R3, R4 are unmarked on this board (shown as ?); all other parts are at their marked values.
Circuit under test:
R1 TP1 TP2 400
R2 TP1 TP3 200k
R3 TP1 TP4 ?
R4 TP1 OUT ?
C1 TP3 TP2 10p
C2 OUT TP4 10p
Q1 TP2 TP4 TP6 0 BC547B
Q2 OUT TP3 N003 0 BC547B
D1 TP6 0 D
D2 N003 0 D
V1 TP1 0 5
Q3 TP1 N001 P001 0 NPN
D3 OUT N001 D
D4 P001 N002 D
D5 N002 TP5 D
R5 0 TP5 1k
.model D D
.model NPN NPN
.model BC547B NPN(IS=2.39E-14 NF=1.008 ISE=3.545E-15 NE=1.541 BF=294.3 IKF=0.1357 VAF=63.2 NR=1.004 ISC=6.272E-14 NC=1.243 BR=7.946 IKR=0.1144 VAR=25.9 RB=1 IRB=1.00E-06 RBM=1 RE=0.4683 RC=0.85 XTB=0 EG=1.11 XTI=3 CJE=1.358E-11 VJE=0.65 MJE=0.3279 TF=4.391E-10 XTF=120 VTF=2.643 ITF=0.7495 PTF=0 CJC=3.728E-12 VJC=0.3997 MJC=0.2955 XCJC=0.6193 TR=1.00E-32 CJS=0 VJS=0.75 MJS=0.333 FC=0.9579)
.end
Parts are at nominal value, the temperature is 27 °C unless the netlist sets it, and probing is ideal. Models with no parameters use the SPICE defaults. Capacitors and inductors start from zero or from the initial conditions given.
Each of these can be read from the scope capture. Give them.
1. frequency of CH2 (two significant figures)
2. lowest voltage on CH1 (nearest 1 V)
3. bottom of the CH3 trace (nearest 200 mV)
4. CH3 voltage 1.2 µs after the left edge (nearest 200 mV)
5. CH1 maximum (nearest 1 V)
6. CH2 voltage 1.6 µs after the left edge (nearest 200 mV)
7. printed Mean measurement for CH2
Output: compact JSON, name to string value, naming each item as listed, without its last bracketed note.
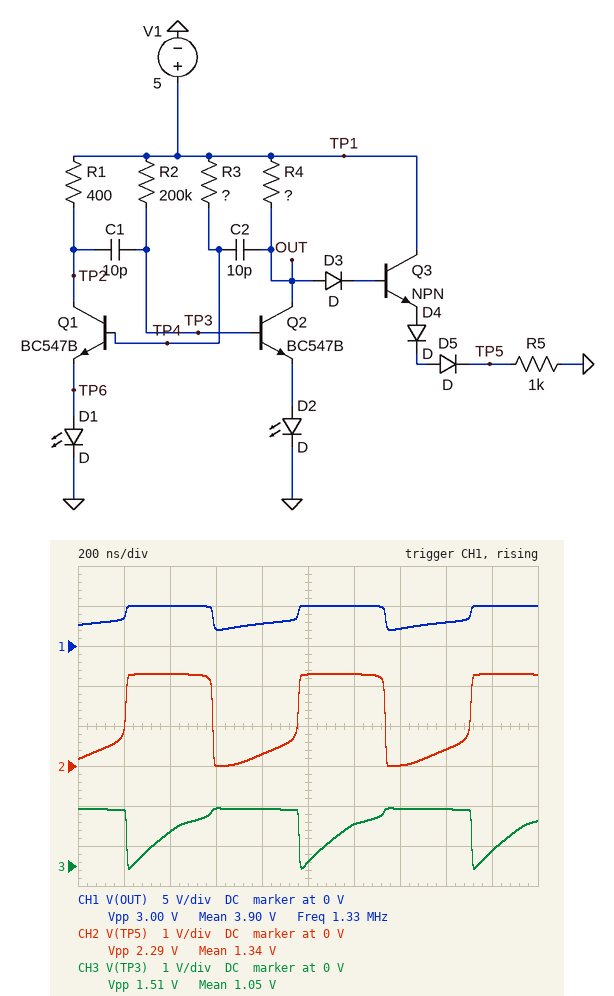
{"frequency of CH2": "1.3 MHz", "lowest voltage on CH1": "2 V", "bottom of the CH3 trace": "0 V", "CH3 voltage 1.2 µs after the left edge": "1.0 V", "CH1 maximum": "5 V", "CH2 voltage 1.6 µs after the left edge": "400 mV", "printed Mean measurement for CH2": "1.34 V"}
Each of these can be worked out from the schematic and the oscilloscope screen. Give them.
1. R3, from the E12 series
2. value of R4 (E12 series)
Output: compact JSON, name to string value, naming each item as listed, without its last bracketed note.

{"R3, from the E12 series": "330 kΩ", "value of R4": "220 Ω"}
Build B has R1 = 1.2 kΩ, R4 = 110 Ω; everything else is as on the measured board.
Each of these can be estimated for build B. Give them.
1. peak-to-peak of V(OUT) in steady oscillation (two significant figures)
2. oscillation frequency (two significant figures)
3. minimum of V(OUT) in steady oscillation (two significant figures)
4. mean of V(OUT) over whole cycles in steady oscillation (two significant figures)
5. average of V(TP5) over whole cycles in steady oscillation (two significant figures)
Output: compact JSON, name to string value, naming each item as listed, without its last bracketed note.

{"peak-to-peak of V(OUT) in steady oscillation": "3.5 V", "oscillation frequency": "770 kHz", "minimum of V(OUT) in steady oscillation": "1.5 V", "mean of V(OUT) over whole cycles in steady oscillation": "4.5 V", "average of V(TP5) over whole cycles in steady oscillation": "1.9 V"}
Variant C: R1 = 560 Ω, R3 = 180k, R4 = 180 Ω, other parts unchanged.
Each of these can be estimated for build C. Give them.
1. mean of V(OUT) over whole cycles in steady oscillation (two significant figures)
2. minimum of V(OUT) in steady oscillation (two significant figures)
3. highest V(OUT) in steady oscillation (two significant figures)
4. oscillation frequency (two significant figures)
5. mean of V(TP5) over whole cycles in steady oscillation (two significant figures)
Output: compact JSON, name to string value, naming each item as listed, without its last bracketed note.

{"mean of V(OUT) over whole cycles in steady oscillation": "4.1 V", "minimum of V(OUT) in steady oscillation": "930 mV", "highest V(OUT) in steady oscillation": "5.0 V", "oscillation frequency": "890 kHz", "mean of V(TP5) over whole cycles in steady oscillation": "1.7 V"}
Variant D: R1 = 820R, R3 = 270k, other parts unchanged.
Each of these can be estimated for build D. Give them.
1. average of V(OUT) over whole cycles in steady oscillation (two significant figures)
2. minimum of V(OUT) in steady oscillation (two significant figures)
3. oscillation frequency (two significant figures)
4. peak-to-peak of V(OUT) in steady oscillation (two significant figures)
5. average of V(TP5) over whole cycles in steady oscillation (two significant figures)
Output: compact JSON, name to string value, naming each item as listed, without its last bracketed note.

{"average of V(OUT) over whole cycles in steady oscillation": "3.9 V", "minimum of V(OUT) in steady oscillation": "860 mV", "oscillation frequency": "730 kHz", "peak-to-peak of V(OUT) in steady oscillation": "4.1 V", "average of V(TP5) over whole cycles in steady oscillation": "1.6 V"}
